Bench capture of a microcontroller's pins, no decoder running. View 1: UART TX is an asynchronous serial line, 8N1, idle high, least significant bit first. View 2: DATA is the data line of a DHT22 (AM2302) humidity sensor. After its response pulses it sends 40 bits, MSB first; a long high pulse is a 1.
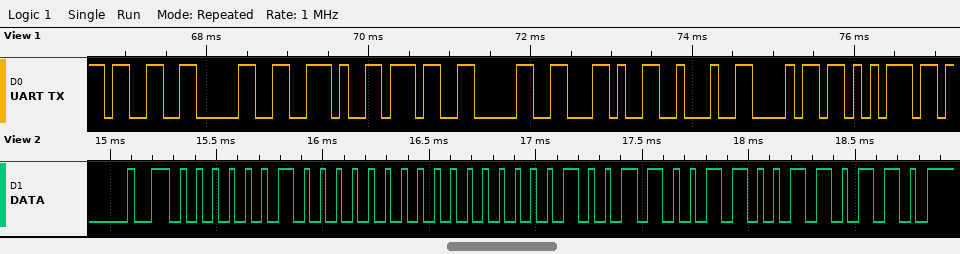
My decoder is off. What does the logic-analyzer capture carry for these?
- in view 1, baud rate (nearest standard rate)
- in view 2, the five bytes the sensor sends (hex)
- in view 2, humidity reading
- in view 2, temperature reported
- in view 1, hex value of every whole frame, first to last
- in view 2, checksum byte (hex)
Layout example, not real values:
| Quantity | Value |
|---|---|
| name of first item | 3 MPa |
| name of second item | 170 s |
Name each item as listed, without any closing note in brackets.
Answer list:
| Quantity | Value |
|---|---|
| in view 1, baud rate | 9600 baud |
| in view 2, the five bytes the sensor sends | 02 00 01 33 36 |
| in view 2, humidity reading | 51.2 % |
| in view 2, temperature reported | 30.7 °C |
| in view 1, hex value of every whole frame, first to last | 0x33 0x30 0x2E 0x37 0x30 0x2C 0x22 0x68 0x75 |
| in view 2, checksum byte | 0x36 |
